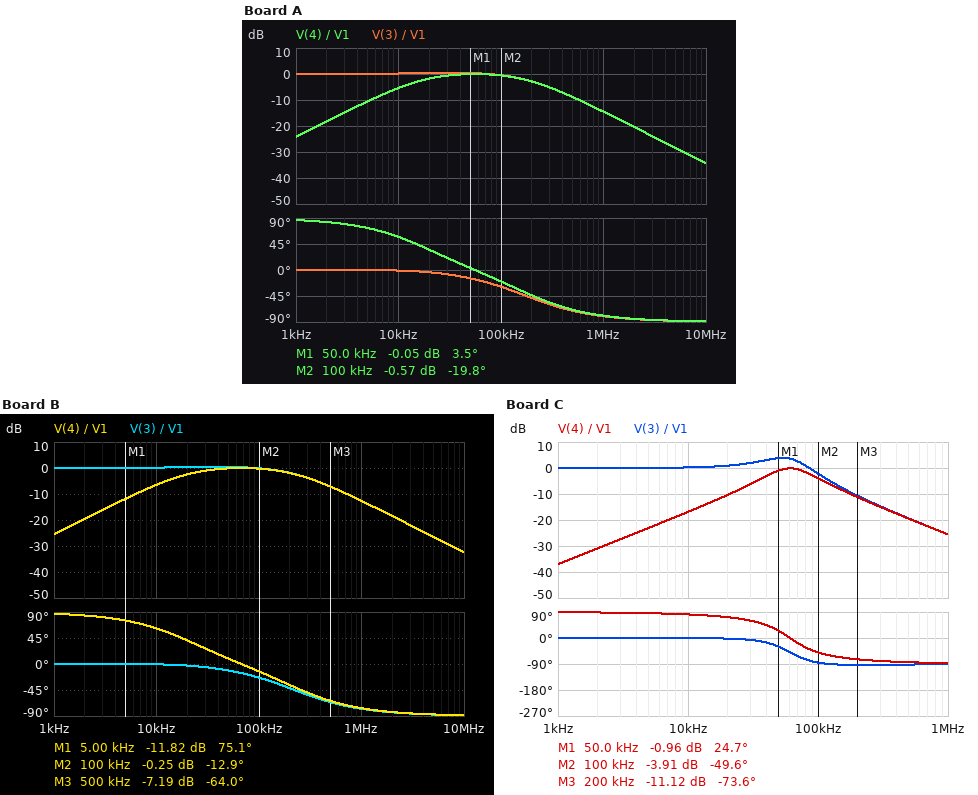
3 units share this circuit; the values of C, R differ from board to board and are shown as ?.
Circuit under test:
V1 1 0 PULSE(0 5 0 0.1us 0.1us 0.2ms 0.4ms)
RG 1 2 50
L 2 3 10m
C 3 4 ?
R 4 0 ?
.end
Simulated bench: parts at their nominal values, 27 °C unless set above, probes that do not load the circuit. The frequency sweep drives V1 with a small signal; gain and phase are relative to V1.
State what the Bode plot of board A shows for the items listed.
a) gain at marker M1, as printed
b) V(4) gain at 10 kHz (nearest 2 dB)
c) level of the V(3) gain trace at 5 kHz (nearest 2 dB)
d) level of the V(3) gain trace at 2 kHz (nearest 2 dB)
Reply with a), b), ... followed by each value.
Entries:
a) -0.05 dB
b) -6 dB
c) 0 dB
d) 0 dB
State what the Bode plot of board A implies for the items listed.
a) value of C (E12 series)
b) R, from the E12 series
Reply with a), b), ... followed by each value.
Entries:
a) 820 pF
b) 12 kΩ
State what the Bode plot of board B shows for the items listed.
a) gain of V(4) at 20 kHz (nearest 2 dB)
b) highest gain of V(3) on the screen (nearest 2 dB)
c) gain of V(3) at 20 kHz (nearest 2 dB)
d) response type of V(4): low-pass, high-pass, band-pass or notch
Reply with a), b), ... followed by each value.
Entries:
a) -2 dB
b) 0 dB
c) 0 dB
d) band-pass
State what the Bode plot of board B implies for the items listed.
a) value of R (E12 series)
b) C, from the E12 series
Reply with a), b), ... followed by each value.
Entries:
a) 15 kΩ
b) 560 pF
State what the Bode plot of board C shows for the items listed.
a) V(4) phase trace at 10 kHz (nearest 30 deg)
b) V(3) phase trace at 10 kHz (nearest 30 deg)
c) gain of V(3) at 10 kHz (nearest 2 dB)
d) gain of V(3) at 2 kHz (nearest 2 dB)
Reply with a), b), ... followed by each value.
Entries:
a) 90 deg
b) 0 deg
c) 0 dB
d) 0 dB
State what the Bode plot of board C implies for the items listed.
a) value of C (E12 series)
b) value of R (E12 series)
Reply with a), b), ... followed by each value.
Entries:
a) 680 pF
b) 3.3 kΩ
